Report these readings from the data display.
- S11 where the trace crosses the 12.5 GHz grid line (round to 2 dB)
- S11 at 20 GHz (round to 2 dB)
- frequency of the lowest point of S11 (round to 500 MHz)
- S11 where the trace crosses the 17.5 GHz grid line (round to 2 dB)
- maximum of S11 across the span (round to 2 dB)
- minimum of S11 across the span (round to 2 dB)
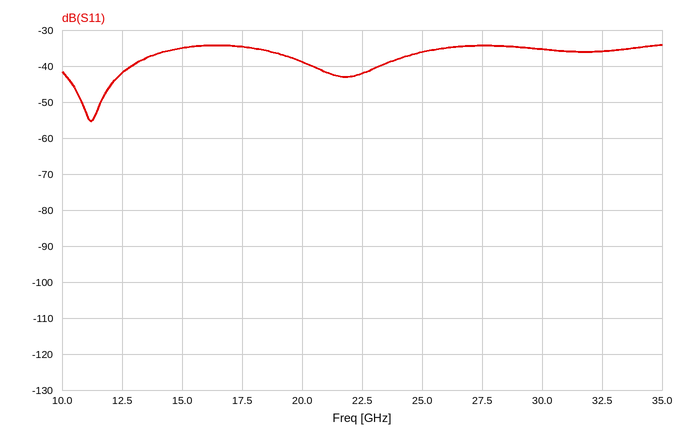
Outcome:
-42 dB
-38 dB
11.0 GHz
-34 dB
-34 dB
-56 dB
